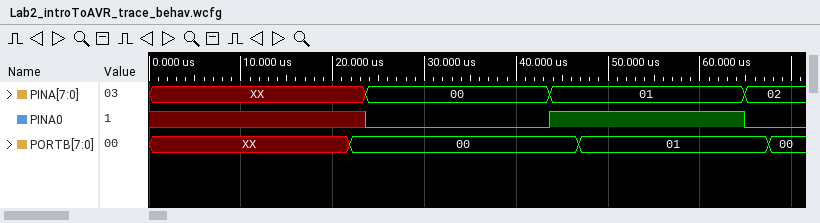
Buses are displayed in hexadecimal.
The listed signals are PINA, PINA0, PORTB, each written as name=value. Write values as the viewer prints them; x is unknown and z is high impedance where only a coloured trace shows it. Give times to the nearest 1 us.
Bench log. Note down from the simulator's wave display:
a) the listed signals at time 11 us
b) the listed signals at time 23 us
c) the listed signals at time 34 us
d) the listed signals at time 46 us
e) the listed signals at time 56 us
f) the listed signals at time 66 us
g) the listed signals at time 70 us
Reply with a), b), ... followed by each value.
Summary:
a) PINA=XX, PINA0=x, PORTB=XX
b) PINA=XX, PINA0=x, PORTB=00
c) PINA=00, PINA0=0, PORTB=00
d) PINA=01, PINA0=1, PORTB=00
e) PINA=01, PINA0=1, PORTB=01
f) PINA=02, PINA0=0, PORTB=01
g) PINA=02, PINA0=0, PORTB=00
